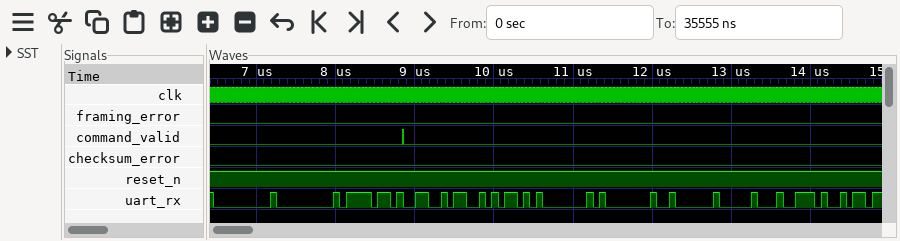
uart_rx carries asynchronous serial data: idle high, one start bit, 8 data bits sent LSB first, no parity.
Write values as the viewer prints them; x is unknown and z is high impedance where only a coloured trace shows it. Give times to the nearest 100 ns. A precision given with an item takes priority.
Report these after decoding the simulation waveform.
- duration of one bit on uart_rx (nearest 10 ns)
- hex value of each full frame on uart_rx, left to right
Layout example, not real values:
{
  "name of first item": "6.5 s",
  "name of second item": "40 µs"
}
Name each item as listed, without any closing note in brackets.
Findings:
{
  "duration of one bit on uart_rx": "80 ns",
  "hex value of each full frame on uart_rx, left to right": "00, 00, 6F, A6, 6A, 01, 01, 02, 10, 2E"
}
